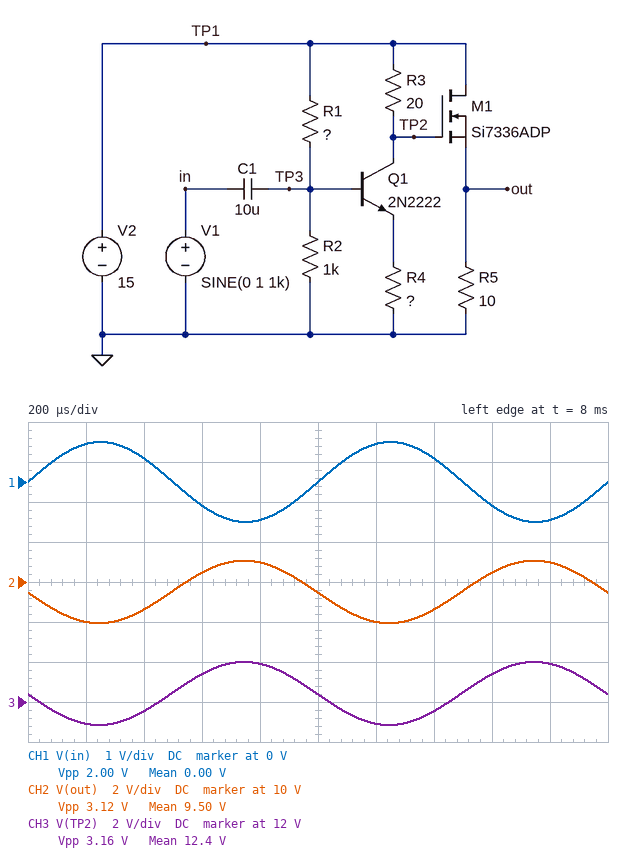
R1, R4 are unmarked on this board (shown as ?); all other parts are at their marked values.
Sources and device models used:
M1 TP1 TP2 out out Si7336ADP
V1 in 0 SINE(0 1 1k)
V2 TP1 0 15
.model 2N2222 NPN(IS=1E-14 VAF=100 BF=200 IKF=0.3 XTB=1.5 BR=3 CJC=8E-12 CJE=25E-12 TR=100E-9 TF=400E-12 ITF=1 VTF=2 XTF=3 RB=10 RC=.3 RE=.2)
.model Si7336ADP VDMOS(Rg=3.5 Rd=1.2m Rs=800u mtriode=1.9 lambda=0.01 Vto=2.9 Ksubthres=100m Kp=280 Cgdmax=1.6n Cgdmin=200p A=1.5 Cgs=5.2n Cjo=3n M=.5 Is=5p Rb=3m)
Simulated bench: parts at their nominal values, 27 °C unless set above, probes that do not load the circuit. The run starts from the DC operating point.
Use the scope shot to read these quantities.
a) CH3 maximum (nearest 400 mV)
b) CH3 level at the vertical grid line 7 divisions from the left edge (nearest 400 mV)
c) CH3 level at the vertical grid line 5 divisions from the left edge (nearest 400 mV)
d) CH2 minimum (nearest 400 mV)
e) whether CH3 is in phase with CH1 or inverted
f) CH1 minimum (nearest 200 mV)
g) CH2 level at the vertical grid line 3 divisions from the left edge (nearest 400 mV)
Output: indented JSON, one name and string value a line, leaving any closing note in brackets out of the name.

{
  "CH3 maximum": "14.0 V",
  "CH3 level at the vertical grid line 7 divisions from the left edge": "11.6 V",
  "CH3 level at the vertical grid line 5 divisions from the left edge": "12.4 V",
  "CH2 minimum": "8.0 V",
  "whether CH3 is in phase with CH1 or inverted": "inverted",
  "CH1 minimum": "-1.0 V",
  "CH2 level at the vertical grid line 3 divisions from the left edge": "10.4 V"
}
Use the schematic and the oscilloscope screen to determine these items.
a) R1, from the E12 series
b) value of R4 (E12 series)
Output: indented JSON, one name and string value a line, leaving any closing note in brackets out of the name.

{
  "R1, from the E12 series": "3.9 kΩ",
  "value of R4": "12 Ω"
}
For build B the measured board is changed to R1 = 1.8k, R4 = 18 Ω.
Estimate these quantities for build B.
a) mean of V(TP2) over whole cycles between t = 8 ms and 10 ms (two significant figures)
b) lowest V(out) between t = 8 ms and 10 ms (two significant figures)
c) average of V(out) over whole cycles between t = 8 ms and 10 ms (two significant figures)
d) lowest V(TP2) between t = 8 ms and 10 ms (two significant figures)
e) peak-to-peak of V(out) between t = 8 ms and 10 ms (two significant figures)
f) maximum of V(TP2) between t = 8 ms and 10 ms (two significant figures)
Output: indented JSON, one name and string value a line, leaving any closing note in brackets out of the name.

{
  "mean of V(TP2) over whole cycles between t = 8 ms and 10 ms": "11 V",
  "lowest V(out) between t = 8 ms and 10 ms": "7.1 V",
  "average of V(out) over whole cycles between t = 8 ms and 10 ms": "8.2 V",
  "lowest V(TP2) between t = 8 ms and 10 ms": "10 V",
  "peak-to-peak of V(out) between t = 8 ms and 10 ms": "2.1 V",
  "maximum of V(TP2) between t = 8 ms and 10 ms": "12 V"
}
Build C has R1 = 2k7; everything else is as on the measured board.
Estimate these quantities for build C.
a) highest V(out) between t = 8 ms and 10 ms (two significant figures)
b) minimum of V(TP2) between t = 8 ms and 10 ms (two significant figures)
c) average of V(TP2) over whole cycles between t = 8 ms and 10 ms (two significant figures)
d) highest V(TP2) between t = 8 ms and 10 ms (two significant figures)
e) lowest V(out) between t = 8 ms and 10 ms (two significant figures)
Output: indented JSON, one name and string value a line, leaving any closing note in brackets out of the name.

{
  "highest V(out) between t = 8 ms and 10 ms": "10 V",
  "minimum of V(TP2) between t = 8 ms and 10 ms": "9.8 V",
  "average of V(TP2) over whole cycles between t = 8 ms and 10 ms": "11 V",
  "highest V(TP2) between t = 8 ms and 10 ms": "13 V",
  "lowest V(out) between t = 8 ms and 10 ms": "6.9 V"
}
